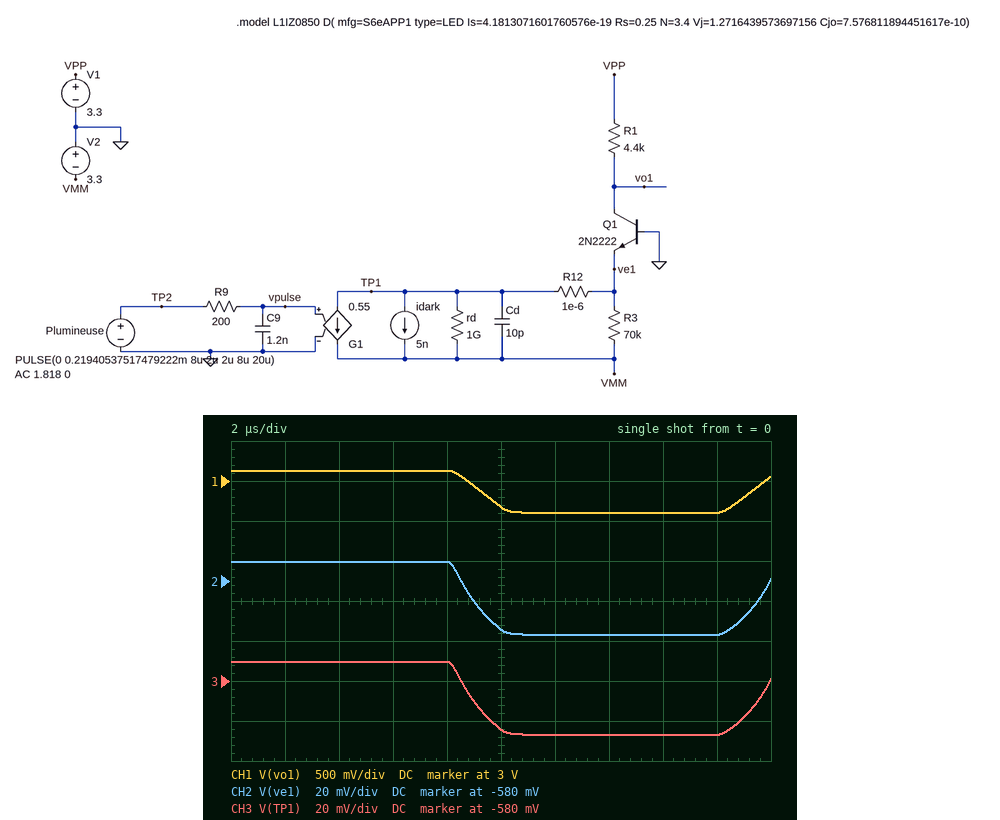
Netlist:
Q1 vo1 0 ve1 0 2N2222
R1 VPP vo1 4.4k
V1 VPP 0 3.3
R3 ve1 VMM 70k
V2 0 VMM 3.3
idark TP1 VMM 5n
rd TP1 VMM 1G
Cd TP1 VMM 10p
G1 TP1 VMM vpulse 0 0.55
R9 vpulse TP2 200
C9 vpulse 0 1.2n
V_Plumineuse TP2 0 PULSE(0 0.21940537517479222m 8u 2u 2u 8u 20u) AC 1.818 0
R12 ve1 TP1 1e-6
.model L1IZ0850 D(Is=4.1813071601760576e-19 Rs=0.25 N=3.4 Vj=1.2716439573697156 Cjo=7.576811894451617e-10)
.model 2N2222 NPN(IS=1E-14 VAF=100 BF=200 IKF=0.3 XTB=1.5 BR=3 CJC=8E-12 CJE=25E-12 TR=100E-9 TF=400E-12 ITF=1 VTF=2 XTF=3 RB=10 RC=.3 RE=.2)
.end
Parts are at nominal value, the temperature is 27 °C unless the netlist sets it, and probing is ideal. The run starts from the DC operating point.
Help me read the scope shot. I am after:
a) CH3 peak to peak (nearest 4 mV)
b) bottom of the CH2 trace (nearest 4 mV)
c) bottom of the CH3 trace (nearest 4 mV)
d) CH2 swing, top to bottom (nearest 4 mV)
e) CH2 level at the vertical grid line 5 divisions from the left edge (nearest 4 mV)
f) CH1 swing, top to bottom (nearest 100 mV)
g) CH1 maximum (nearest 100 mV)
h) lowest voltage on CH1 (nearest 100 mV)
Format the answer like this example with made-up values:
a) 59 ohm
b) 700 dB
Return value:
a) 36 mV
b) -608 mV
c) -608 mV
d) 36 mV
e) -604 mV
f) 500 mV
g) 3.1 V
h) 2.6 V
